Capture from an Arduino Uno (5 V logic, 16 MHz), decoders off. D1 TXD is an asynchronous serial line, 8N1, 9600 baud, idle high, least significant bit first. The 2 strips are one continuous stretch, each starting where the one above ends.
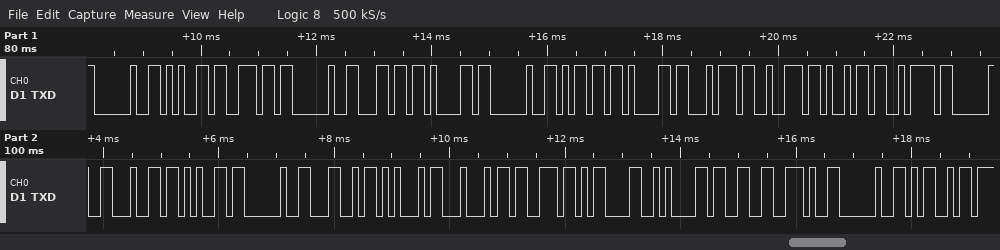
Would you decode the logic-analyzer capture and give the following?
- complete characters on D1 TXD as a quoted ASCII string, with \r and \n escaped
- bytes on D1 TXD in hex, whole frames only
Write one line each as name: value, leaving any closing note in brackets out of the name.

complete characters on D1 TXD as a quoted ASCII string, with \r and \n escaped: " en la matriz de LEDs\r\n3. M"
bytes on D1 TXD in hex, whole frames only: 20 65 6E 20 6C 61 20 6D 61 74 72 69 7A 20 64 65 20 4C 45 44 73 0D 0A 33 2E 20 4D
